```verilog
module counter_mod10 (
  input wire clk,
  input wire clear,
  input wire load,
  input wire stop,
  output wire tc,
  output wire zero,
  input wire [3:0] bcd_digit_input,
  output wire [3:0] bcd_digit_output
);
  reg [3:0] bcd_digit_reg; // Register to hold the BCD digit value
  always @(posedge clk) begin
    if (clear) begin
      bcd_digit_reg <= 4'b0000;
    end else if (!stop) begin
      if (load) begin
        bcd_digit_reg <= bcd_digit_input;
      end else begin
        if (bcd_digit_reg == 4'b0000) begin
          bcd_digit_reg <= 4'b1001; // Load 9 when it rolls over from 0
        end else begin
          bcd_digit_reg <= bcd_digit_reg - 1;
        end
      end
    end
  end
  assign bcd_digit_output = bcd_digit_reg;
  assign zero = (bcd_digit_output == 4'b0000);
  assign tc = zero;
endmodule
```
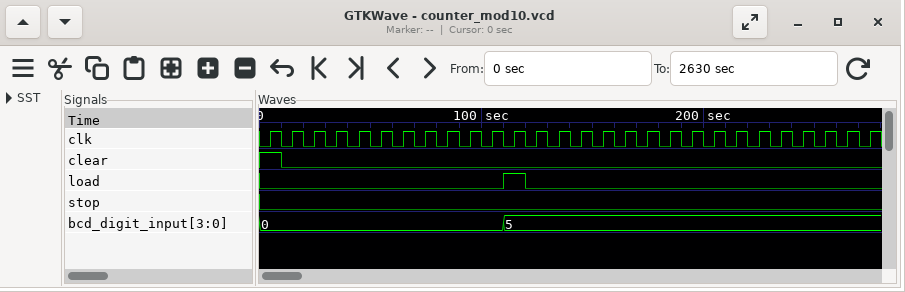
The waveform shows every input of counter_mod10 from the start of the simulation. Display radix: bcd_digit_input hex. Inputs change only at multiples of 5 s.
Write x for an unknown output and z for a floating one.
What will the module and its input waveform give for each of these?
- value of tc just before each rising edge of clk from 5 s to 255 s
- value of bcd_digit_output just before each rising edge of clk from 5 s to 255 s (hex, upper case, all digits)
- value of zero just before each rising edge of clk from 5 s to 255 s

x 1 0 0 0 0 0 0 0 0 0 1 0 0 0 0 0 1 0 0 0 0 0 0 0 0
x, 0, 9, 8, 7, 6, 5, 4, 3, 2, 1, 0, 5, 4, 3, 2, 1, 0, 9, 8, 7, 6, 5, 4, 3, 2
x 1 0 0 0 0 0 0 0 0 0 1 0 0 0 0 0 1 0 0 0 0 0 0 0 0
